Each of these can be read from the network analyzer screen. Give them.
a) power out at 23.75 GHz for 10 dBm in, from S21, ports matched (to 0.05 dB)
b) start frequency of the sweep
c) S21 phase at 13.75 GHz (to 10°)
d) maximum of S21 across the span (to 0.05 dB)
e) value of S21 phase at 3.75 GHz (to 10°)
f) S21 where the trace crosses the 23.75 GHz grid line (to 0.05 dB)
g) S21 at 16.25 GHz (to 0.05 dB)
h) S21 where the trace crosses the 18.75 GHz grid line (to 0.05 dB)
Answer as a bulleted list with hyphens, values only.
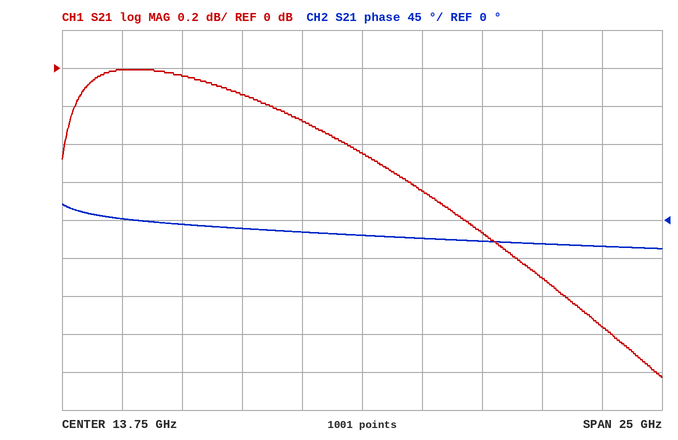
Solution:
- 8.65 dBm
- 1.25 GHz
- -20°
- 0.00 dB
- 0°
- -1.35 dB
- -0.65 dB
- -0.85 dB
